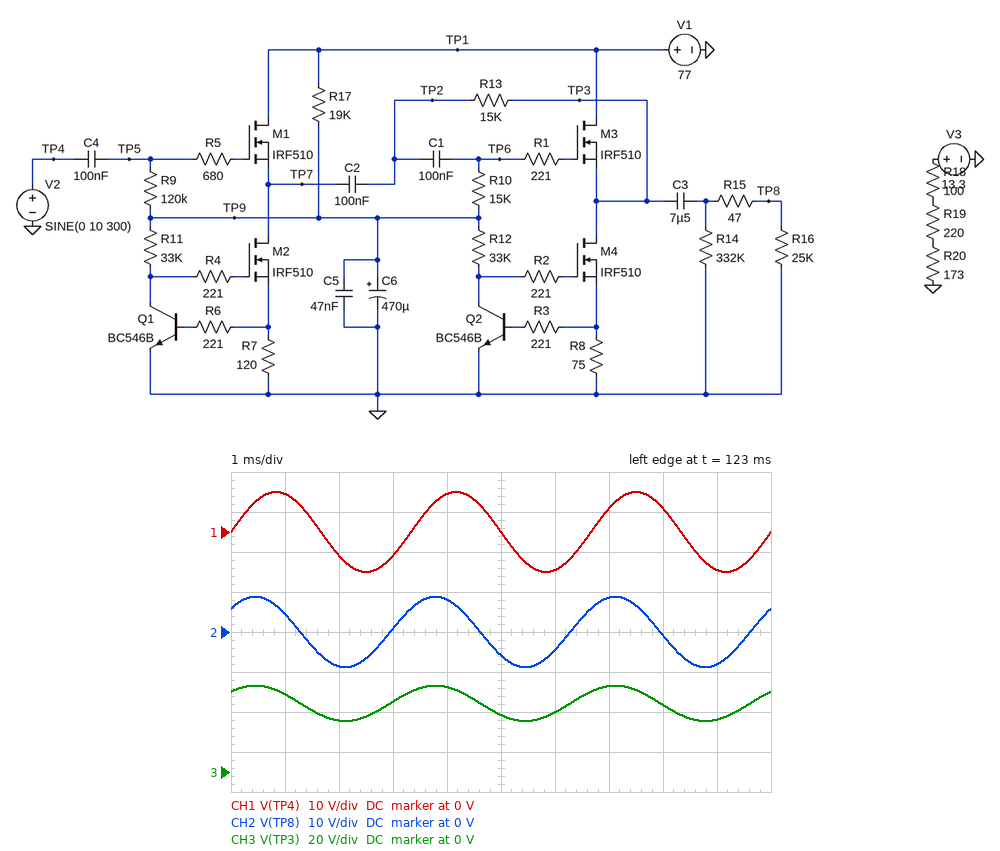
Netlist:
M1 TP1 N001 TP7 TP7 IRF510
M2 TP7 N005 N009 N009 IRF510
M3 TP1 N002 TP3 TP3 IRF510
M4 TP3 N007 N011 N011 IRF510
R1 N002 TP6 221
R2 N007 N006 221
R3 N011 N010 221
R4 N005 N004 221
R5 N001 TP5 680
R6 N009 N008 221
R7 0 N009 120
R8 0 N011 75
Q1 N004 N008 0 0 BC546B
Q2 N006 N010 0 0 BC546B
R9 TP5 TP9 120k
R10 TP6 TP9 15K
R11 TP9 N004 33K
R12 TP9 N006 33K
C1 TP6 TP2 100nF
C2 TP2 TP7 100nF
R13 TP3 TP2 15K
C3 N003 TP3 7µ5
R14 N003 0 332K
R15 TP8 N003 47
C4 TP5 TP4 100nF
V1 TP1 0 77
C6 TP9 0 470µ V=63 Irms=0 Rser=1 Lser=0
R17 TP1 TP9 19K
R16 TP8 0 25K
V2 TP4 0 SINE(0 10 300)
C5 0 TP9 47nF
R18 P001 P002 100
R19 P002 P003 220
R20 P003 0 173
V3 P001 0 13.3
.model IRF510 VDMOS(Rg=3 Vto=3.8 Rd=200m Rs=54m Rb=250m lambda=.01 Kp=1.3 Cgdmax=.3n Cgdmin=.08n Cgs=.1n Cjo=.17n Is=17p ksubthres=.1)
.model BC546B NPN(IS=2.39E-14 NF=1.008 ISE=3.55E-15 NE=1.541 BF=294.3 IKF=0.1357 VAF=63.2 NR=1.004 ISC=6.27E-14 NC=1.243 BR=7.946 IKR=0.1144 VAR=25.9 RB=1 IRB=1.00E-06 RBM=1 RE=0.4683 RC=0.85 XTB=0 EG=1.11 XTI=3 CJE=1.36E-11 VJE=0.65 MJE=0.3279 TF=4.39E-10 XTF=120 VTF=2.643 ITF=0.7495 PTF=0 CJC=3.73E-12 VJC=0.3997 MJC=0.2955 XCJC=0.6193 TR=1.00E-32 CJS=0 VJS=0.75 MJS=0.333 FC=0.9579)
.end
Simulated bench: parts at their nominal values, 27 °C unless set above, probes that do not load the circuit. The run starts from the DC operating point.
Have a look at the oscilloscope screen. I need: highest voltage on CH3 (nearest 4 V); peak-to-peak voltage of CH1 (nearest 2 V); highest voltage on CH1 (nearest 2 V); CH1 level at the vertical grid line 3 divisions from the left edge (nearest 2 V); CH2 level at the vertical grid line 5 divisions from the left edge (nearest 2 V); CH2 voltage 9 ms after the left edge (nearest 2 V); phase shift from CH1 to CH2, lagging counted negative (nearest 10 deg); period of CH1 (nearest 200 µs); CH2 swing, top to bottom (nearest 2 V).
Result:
44 V
20 V
10 V
-6 V
-6 V
-8 V
40 deg
3.4 ms
18 V
